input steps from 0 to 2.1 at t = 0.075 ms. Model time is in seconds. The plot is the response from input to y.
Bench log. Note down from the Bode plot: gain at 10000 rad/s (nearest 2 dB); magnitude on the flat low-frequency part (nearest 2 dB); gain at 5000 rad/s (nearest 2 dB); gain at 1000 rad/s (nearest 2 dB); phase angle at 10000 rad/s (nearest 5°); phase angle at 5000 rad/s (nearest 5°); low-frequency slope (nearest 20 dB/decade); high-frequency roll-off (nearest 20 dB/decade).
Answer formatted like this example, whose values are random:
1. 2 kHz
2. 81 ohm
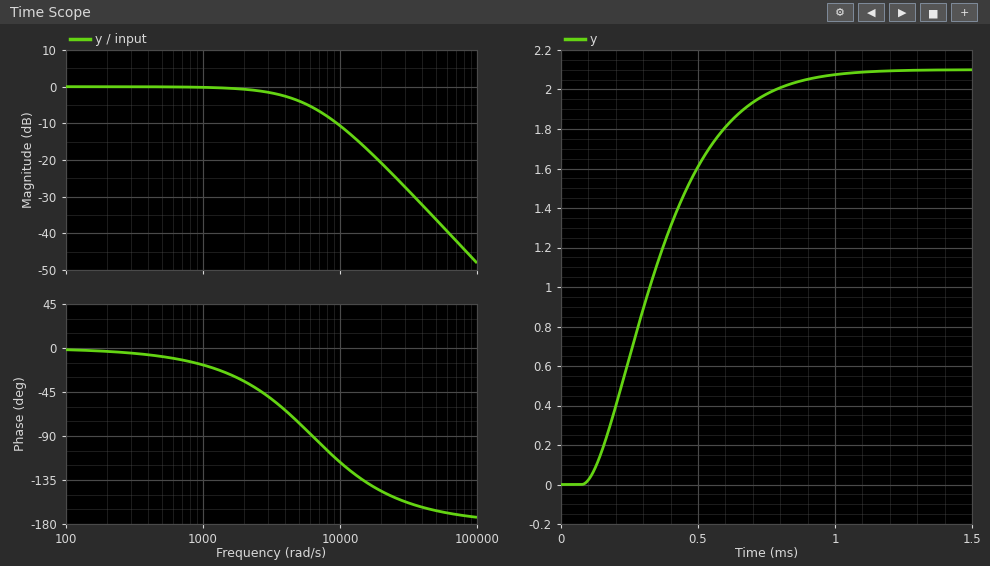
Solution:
1. -10 dB
2. 0 dB
3. -4 dB
4. 0 dB
5. -115°
6. -75°
7. 0 dB/decade
8. -40 dB/decade
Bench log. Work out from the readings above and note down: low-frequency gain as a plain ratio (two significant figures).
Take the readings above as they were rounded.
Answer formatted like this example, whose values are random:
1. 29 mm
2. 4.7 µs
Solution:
1. 1.0
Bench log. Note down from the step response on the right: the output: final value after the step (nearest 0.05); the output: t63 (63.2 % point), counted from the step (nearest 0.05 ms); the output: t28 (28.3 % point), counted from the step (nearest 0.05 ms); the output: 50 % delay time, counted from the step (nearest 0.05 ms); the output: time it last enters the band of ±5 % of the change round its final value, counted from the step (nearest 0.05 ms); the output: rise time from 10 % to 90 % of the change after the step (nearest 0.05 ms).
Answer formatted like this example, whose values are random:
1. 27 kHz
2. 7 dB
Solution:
1. 2.10
2. 0.35 ms
3. 0.15 ms
4. 0.25 ms
5. 0.70 ms
6. 0.50 ms
